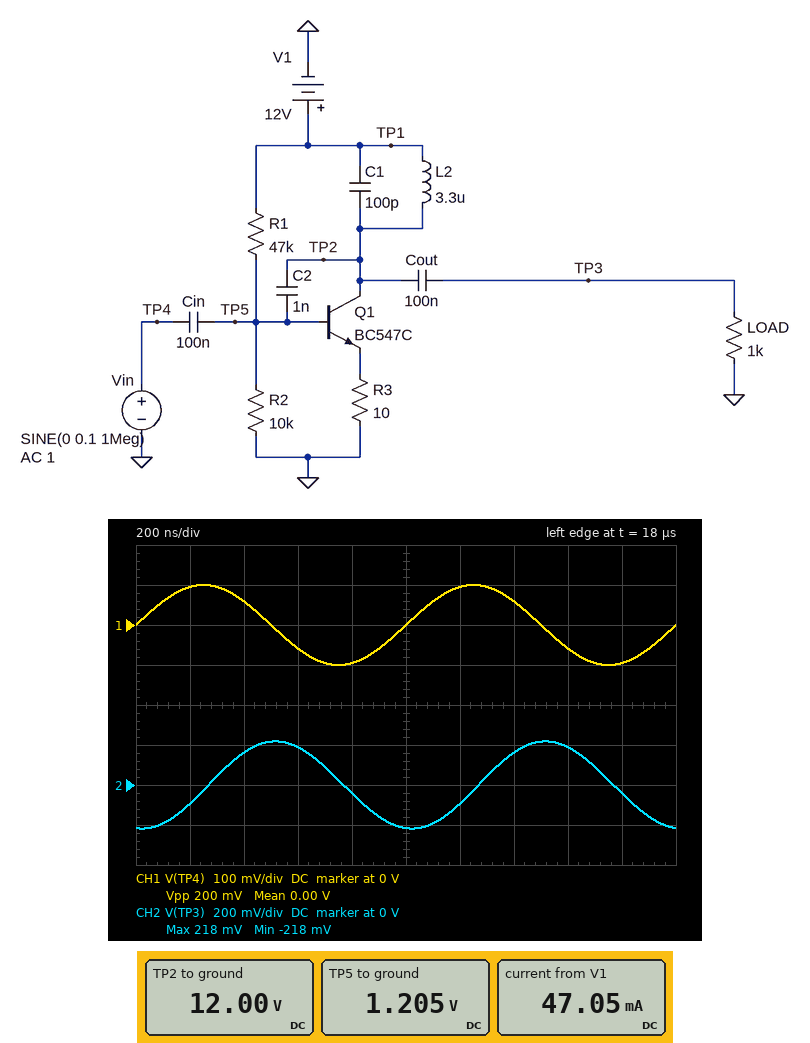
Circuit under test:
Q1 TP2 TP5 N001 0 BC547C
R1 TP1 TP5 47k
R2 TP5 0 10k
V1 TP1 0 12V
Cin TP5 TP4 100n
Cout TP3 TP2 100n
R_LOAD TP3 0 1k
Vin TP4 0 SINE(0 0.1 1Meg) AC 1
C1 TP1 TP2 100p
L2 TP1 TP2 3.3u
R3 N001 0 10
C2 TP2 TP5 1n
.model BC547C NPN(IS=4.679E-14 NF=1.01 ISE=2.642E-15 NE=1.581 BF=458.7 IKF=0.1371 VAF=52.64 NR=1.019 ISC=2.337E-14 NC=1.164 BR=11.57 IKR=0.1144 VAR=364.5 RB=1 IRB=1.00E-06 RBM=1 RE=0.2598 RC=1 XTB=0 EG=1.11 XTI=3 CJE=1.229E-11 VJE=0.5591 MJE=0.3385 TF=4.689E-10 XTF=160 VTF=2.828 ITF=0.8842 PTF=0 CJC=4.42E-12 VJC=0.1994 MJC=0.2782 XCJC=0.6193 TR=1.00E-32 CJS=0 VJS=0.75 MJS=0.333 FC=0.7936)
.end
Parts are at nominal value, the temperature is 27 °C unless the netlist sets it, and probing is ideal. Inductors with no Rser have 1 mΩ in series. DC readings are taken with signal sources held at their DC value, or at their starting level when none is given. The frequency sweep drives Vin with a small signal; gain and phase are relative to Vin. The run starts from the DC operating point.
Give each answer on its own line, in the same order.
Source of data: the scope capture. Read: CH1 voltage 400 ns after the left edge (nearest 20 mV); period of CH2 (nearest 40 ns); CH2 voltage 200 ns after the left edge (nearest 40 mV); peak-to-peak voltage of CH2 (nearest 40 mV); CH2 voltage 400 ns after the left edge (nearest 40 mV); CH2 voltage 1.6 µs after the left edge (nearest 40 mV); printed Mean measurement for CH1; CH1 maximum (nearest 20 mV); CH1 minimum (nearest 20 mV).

60 mV
1.00 µs
-80 mV
440 mV
160 mV
200 mV
0.00 V
100 mV
-100 mV
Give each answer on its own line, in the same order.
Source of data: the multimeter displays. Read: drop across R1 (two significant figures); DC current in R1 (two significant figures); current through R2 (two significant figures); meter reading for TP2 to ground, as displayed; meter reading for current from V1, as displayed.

11 V
230 µA
120 µA
12.00 V
47.05 mA
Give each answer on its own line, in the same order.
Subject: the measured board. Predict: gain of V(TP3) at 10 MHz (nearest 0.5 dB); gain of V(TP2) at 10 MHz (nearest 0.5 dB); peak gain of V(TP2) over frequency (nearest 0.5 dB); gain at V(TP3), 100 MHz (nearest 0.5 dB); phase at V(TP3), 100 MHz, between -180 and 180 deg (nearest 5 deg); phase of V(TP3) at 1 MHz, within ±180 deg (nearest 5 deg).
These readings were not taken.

5.0 dB
5.0 dB
33.5 dB
-0.5 dB
5 deg
-95 deg
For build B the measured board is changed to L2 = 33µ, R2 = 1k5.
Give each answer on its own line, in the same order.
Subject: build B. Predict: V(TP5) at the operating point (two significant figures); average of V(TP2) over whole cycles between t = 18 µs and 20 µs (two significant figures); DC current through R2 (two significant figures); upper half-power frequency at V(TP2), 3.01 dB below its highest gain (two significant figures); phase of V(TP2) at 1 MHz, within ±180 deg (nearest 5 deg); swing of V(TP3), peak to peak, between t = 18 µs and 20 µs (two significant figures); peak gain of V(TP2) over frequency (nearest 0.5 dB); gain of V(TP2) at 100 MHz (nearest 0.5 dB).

370 mV
12 V
250 µA
930 kHz
25 deg
550 mV
14.5 dB
-1.0 dB
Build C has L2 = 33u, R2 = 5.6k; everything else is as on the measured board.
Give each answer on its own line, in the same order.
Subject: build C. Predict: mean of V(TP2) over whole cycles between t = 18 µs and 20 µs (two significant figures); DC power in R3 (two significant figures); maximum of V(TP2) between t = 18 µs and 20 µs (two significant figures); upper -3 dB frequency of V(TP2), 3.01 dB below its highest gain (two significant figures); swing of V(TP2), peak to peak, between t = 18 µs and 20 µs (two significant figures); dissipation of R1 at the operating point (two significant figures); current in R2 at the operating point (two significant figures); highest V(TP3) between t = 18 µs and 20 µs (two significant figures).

12 V
7.5 mW
15 V
990 kHz
6.2 V
2.6 mW
180 µA
3.1 V
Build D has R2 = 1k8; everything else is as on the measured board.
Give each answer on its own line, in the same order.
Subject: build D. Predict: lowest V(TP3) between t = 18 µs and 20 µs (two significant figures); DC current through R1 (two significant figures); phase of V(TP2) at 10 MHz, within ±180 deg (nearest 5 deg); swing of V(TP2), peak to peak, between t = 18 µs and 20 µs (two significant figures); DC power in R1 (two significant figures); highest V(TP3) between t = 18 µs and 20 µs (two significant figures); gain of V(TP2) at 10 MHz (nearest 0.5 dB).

-16 mV
250 µA
0 deg
32 mV
2.8 mW
16 mV
0 dB
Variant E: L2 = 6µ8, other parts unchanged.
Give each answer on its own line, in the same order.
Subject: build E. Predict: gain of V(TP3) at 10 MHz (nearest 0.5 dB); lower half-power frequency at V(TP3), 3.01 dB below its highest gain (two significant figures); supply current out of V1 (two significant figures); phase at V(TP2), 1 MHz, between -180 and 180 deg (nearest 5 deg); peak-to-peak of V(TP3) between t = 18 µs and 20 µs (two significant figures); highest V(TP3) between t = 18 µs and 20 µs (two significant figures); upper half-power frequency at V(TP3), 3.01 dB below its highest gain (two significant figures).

4.5 dB
1.7 MHz
47 mA
-100 deg
1.1 V
550 mV
2.0 MHz
